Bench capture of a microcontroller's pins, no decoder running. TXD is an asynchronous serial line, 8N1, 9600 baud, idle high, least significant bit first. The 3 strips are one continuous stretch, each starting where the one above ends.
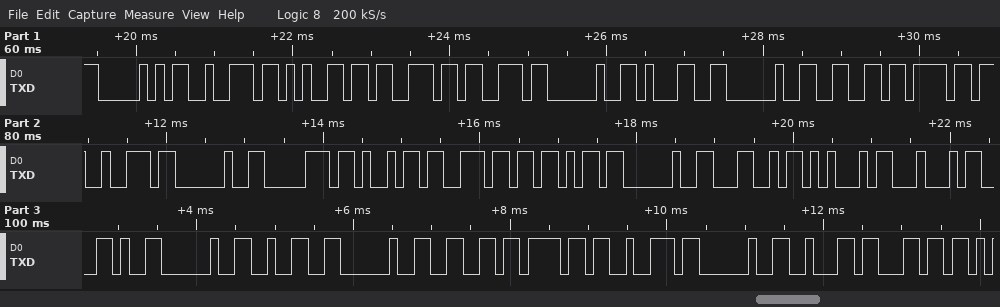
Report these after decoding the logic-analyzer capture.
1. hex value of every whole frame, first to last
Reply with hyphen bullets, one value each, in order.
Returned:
- 50 72 65 73 73 20 31 20 66 6F 72 20 70 69 6E 6B 20 4C 45 44 2C 20 32 20 66 6F 72 20 62 6C
